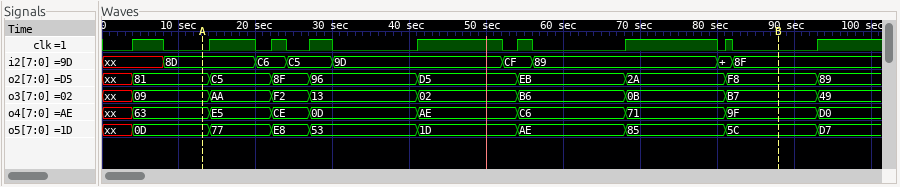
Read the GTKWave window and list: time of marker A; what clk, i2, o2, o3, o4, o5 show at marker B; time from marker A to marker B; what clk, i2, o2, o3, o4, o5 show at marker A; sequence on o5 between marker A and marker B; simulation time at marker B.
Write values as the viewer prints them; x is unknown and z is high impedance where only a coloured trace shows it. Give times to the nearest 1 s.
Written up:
13 s
clk=0, i2=8F, o2=F8, o3=B7, o4=9F, o5=5C
75 s
clk=0, i2=8D, o2=81, o3=09, o4=63, o5=0D
0D, 77, E8, 53, 1D, AE, 85, 5C
88 s
